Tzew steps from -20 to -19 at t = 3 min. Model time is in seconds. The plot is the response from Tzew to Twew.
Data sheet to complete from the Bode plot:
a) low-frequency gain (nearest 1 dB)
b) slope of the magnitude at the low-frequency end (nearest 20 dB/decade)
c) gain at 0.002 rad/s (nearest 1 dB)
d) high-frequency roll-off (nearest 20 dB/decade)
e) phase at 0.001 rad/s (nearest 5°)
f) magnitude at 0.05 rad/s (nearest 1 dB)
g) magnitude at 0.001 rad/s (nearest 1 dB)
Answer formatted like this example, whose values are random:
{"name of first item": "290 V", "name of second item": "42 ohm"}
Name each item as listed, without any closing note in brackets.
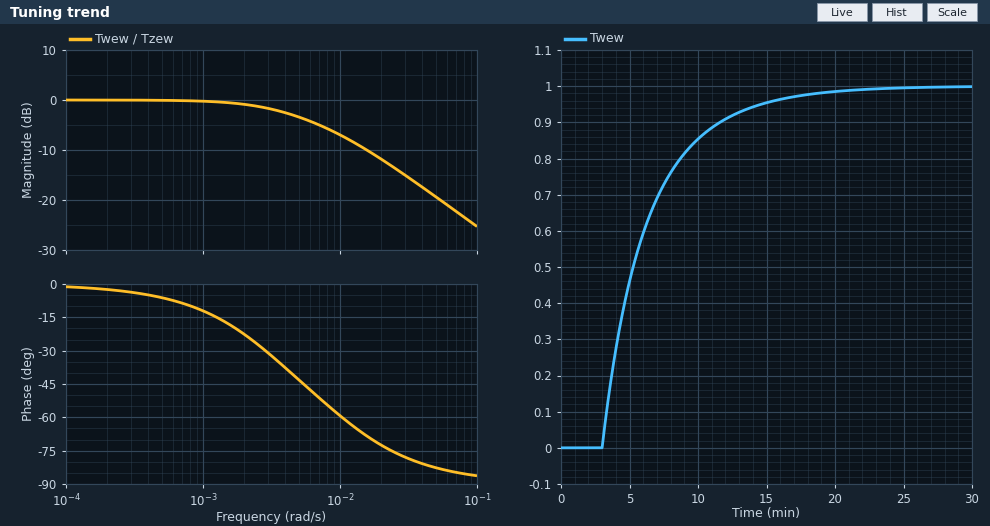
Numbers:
{"low-frequency gain": "0 dB", "slope of the magnitude at the low-frequency end": "0 dB/decade", "gain at 0.002 rad/s": "-1 dB", "high-frequency roll-off": "-20 dB/decade", "phase at 0.001 rad/s": "-10°", "magnitude at 0.05 rad/s": "-19 dB", "magnitude at 0.001 rad/s": "0 dB"}
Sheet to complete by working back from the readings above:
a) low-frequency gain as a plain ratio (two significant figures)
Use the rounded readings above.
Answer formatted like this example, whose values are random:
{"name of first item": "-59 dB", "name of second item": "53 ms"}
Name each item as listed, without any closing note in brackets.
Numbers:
{"low-frequency gain as a plain ratio": "1.0"}
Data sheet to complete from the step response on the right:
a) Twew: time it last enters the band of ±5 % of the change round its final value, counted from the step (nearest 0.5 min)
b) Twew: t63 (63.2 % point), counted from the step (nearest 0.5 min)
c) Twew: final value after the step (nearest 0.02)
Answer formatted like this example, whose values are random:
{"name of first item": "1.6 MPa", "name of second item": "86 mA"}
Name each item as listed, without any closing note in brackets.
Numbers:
{"Twew: time it last enters the band of ±5 % of the change round its final value, counted from the step": "11.5 min", "Twew: t63 (63.2 % point), counted from the step": "3.5 min", "Twew: final value after the step": "1.00"}
